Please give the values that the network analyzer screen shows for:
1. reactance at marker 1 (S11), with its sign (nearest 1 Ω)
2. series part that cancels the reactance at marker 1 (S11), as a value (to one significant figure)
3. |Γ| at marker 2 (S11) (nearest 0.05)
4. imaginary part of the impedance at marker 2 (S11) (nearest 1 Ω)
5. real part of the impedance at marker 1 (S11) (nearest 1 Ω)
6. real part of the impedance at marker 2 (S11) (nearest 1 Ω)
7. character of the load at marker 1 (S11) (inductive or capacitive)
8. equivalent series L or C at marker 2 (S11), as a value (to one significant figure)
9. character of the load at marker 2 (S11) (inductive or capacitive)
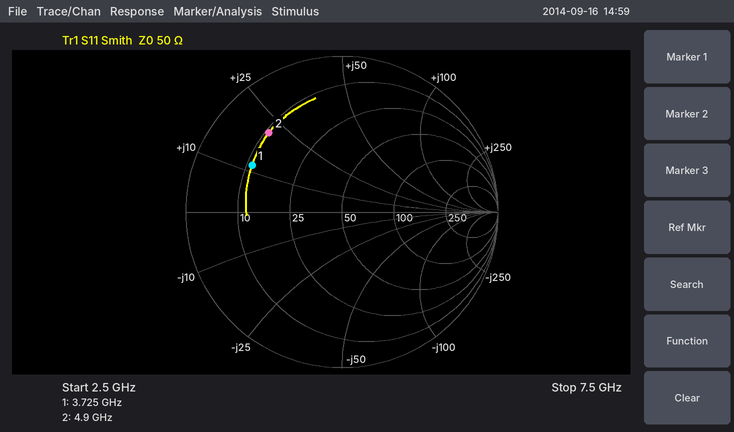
+12 Ω
4 pF
0.70
+21 Ω
11 Ω
11 Ω
inductive
700 pH
inductive
